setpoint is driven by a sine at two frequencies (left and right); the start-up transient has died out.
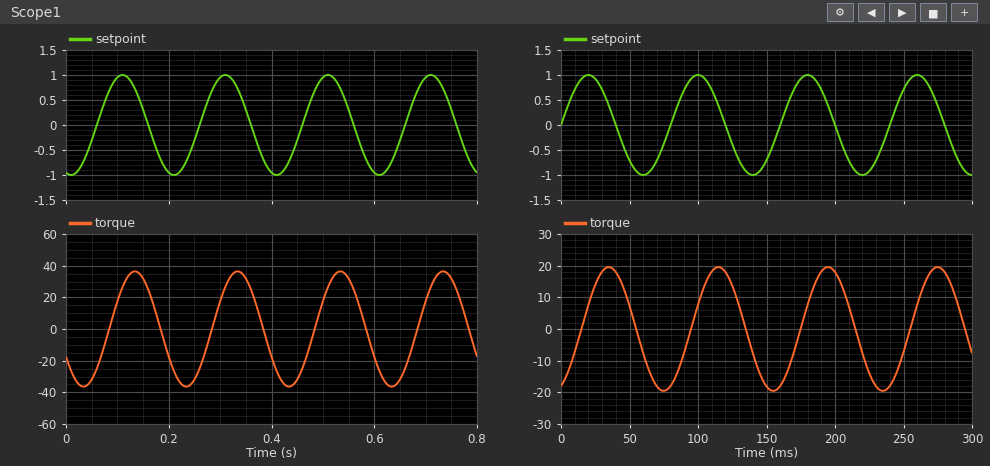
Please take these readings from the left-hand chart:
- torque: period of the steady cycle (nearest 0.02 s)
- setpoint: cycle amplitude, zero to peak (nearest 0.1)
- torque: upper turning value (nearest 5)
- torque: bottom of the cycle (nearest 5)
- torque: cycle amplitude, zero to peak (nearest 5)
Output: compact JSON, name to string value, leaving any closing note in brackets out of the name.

{"torque: period of the steady cycle": "0.20 s", "setpoint: cycle amplitude, zero to peak": "1.0", "torque: upper turning value": "35", "torque: bottom of the cycle": "-35", "torque: cycle amplitude, zero to peak": "35"}
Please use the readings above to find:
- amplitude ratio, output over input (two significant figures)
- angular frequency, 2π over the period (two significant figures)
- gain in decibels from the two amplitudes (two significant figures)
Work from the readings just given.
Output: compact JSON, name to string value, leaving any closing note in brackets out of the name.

{"amplitude ratio, output over input": "35", "angular frequency, 2π over the period": "31 rad/s", "gain in decibels from the two amplitudes": "31 dB"}
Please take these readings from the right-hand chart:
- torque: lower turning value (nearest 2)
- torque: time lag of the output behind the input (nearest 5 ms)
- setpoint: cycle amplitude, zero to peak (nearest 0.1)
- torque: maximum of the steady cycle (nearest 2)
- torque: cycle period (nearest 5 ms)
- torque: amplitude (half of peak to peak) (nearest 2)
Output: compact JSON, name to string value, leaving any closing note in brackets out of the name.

{"torque: lower turning value": "-20", "torque: time lag of the output behind the input": "15 ms", "setpoint: cycle amplitude, zero to peak": "1.0", "torque: maximum of the steady cycle": "20", "torque: cycle period": "80 ms", "torque: amplitude (half of peak to peak)": "20"}
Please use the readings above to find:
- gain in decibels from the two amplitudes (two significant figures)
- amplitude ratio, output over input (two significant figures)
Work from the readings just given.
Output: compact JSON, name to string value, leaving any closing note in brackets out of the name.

{"gain in decibels from the two amplitudes": "26 dB", "amplitude ratio, output over input": "20"}
